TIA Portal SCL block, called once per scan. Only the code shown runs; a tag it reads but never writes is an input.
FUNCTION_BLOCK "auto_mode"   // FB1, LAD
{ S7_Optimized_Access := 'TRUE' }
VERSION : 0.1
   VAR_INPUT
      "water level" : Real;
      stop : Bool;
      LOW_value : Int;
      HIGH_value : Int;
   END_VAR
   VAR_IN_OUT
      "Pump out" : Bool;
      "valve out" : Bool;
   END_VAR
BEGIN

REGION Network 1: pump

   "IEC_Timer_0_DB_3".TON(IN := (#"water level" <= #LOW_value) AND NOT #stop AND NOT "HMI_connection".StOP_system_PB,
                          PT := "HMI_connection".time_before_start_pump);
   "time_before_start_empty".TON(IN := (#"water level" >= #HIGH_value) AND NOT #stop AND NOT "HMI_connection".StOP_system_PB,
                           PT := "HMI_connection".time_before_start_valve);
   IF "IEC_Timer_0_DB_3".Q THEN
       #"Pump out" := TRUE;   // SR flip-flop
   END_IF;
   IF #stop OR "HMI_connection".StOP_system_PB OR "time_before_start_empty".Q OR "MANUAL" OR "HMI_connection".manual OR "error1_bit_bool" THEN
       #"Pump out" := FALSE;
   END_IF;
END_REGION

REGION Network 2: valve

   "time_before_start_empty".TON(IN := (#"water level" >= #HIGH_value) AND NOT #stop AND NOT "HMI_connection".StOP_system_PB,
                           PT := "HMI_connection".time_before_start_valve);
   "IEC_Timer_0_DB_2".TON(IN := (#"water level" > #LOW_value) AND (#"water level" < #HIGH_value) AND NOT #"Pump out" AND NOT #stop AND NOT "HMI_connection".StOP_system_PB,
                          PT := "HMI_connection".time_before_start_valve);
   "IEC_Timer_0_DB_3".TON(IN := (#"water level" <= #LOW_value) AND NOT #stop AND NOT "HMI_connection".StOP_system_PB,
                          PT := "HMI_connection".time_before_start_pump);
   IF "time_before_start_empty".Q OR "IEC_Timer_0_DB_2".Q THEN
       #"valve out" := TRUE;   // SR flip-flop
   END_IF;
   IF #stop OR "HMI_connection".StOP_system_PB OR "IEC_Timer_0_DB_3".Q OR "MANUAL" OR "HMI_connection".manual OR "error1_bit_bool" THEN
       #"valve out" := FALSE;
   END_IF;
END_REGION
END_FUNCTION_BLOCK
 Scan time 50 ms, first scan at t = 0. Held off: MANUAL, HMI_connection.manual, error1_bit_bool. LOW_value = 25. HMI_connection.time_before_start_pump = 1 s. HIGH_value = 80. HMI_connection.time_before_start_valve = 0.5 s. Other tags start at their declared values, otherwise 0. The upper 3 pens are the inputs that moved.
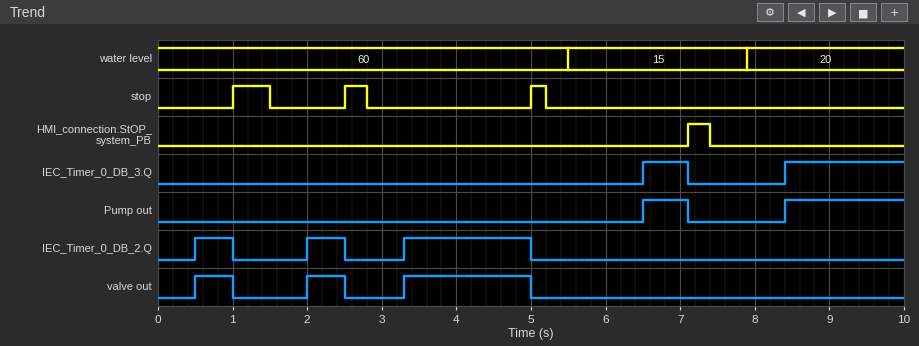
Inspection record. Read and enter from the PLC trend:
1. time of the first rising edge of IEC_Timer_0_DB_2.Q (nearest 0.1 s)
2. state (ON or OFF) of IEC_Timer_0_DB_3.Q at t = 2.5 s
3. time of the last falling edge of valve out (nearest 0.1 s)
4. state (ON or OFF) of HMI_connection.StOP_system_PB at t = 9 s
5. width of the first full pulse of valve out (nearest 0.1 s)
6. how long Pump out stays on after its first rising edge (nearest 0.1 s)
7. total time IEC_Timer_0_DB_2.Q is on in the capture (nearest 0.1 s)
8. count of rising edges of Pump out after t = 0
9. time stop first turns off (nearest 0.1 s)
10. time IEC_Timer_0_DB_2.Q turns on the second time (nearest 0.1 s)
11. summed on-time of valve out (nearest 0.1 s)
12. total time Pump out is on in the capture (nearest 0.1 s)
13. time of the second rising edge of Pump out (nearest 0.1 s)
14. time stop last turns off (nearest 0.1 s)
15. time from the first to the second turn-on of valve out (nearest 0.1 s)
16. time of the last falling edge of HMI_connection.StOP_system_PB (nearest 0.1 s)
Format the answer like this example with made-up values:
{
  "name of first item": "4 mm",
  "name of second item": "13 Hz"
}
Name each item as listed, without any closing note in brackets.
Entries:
{
  "time of the first rising edge of IEC_Timer_0_DB_2.Q": "0.5 s",
  "state (ON or OFF) of IEC_Timer_0_DB_3.Q at t = 2.5 s": "OFF",
  "time of the last falling edge of valve out": "5.0 s",
  "state (ON or OFF) of HMI_connection.StOP_system_PB at t = 9 s": "OFF",
  "width of the first full pulse of valve out": "0.5 s",
  "how long Pump out stays on after its first rising edge": "0.6 s",
  "total time IEC_Timer_0_DB_2.Q is on in the capture": "2.7 s",
  "count of rising edges of Pump out after t = 0": "2",
  "time stop first turns off": "1.5 s",
  "time IEC_Timer_0_DB_2.Q turns on the second time": "2.0 s",
  "summed on-time of valve out": "2.7 s",
  "total time Pump out is on in the capture": "2.2 s",
  "time of the second rising edge of Pump out": "8.4 s",
  "time stop last turns off": "5.2 s",
  "time from the first to the second turn-on of valve out": "1.5 s",
  "time of the last falling edge of HMI_connection.StOP_system_PB": "7.4 s"
}
